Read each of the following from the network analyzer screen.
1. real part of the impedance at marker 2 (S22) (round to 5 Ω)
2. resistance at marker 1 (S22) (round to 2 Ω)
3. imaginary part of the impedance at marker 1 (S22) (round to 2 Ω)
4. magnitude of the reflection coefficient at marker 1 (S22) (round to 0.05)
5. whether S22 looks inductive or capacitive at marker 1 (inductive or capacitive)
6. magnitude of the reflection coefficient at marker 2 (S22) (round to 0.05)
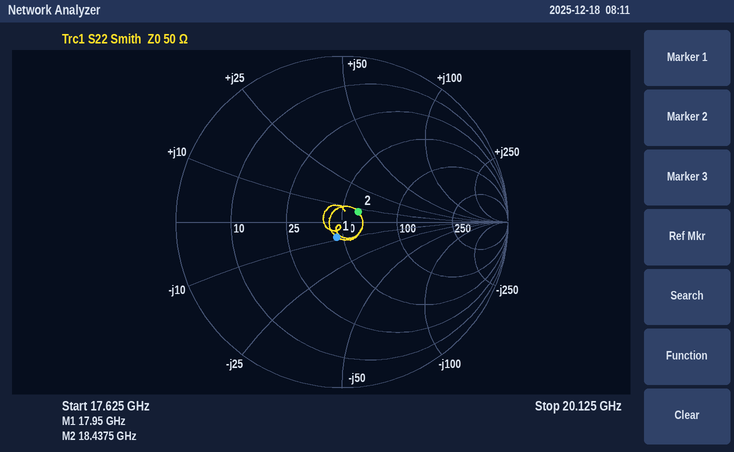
60 Ω
46 Ω
-8 Ω
0.10
capacitive
0.10
